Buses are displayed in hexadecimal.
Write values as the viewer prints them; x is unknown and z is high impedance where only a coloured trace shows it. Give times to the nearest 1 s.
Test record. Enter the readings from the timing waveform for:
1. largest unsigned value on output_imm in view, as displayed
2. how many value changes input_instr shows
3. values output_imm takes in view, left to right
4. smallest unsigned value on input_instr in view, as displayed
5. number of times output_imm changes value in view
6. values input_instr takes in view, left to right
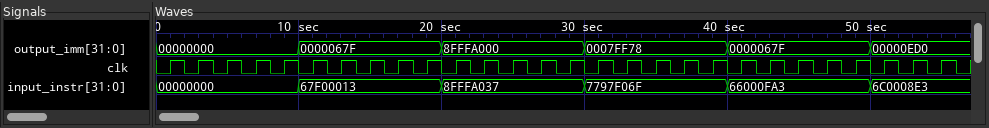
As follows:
8FFFA000
5
00000000, 0000067F, 8FFFA000, 0007FF78, 0000067F, 00000ED0
00000000
5
00000000, 67F00013, 8FFFA037, 7797F06F, 66000FA3, 6C0008E3
